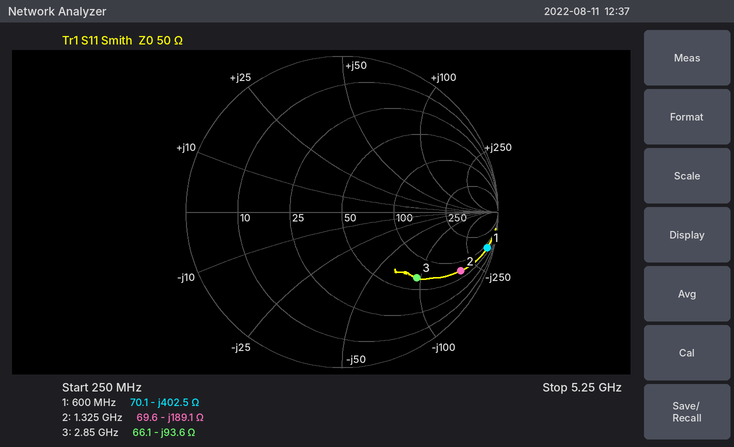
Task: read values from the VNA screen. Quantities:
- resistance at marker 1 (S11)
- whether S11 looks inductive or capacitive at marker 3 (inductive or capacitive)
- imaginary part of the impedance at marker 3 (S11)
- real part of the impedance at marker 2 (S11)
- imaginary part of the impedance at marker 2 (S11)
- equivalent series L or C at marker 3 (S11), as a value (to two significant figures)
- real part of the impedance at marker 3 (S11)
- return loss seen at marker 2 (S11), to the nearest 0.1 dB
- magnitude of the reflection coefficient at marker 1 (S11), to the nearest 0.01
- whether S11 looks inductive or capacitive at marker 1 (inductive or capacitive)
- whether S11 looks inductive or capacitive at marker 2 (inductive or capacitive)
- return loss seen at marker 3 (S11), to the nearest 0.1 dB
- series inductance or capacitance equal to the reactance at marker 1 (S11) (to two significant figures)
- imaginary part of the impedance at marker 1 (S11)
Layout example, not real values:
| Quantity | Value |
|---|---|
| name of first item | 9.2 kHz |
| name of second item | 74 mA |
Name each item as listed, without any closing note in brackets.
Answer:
| Quantity | Value |
|---|---|
| resistance at marker 1 | 70.1 Ω |
| whether S11 looks inductive or capacitive at marker 3 | capacitive |
| imaginary part of the impedance at marker 3 | -93.6 Ω |
| real part of the impedance at marker 2 | 69.6 Ω |
| imaginary part of the impedance at marker 2 | -189.1 Ω |
| equivalent series L or C at marker 3 (S11), as a value | 600 fF |
| real part of the impedance at marker 3 | 66.1 Ω |
| return loss seen at marker 2 (S11), to the nearest 0.1 dB | 1.4 dB |
| magnitude of the reflection coefficient at marker 1 (S11), to the nearest 0.01 | 0.96 |
| whether S11 looks inductive or capacitive at marker 1 | capacitive |
| whether S11 looks inductive or capacitive at marker 2 | capacitive |
| return loss seen at marker 3 (S11), to the nearest 0.1 dB | 3.9 dB |
| series inductance or capacitance equal to the reactance at marker 1 (S11) | 660 fF |
| imaginary part of the impedance at marker 1 | -402.5 Ω |
